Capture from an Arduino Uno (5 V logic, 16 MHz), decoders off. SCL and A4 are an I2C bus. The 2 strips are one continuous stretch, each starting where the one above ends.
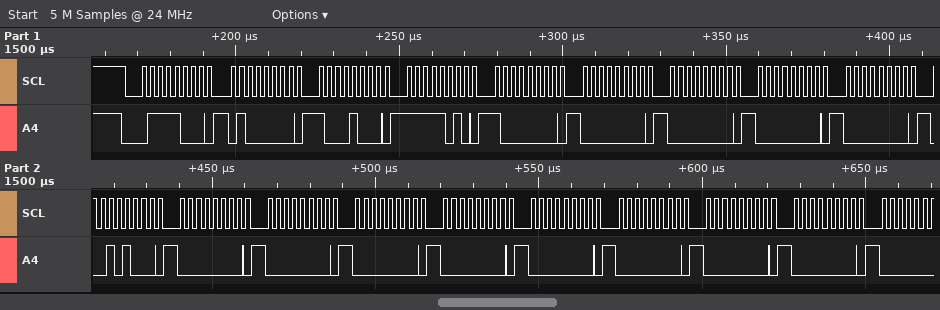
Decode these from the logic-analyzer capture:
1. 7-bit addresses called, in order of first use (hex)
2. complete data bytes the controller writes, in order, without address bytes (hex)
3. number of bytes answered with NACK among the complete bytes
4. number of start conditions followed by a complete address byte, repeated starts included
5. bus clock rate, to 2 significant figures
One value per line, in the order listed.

0x3C
40 88 FA 80 00 00 00 00 28 00 00 00 00 00 00 00 00
0
1
400 kHz
